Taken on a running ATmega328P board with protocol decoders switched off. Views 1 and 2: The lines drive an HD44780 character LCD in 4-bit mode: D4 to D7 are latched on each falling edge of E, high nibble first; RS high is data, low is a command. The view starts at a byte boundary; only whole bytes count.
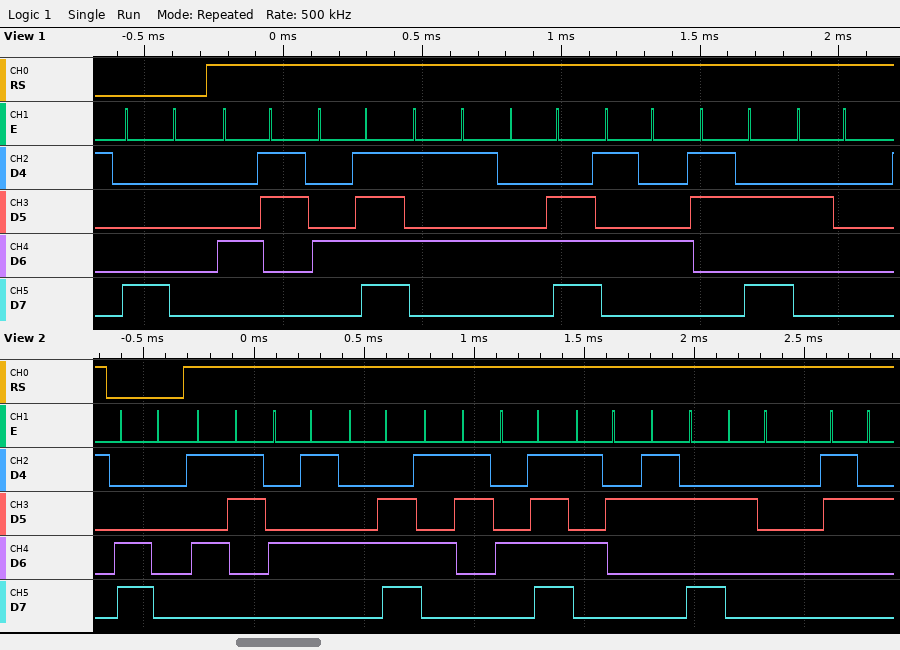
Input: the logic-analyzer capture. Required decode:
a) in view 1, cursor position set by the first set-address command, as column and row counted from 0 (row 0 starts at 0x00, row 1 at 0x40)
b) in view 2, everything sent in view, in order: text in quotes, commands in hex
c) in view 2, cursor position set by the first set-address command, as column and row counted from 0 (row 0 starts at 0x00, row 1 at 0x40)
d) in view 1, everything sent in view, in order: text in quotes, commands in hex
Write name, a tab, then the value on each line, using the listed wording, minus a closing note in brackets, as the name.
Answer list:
in view 1, cursor position set by the first set-address command, as column and row counted from 0	column 0, row 0
in view 2, everything sent in view, in order: text in quotes, commands in hex	0xC0 "SENSOR: 2"
in view 2, cursor position set by the first set-address command, as column and row counted from 0	column 0, row 1
in view 1, everything sent in view, in order: text in quotes, commands in hex	0x80 "COUNT: "
